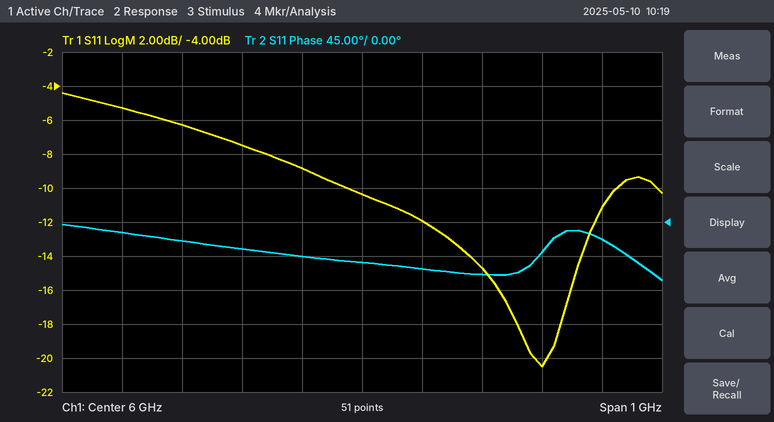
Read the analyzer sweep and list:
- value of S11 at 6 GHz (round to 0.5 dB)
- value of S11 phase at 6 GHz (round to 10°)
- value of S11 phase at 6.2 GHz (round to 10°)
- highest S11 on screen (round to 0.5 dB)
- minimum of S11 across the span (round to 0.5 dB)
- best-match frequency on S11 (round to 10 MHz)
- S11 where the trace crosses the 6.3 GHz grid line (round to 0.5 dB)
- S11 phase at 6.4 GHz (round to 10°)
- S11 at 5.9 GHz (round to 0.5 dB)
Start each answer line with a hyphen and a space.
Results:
- -10.5 dB
- -50°
- -70°
- -4.5 dB
- -20.5 dB
- 6.30 GHz
- -20.5 dB
- -20°
- -9.0 dB
